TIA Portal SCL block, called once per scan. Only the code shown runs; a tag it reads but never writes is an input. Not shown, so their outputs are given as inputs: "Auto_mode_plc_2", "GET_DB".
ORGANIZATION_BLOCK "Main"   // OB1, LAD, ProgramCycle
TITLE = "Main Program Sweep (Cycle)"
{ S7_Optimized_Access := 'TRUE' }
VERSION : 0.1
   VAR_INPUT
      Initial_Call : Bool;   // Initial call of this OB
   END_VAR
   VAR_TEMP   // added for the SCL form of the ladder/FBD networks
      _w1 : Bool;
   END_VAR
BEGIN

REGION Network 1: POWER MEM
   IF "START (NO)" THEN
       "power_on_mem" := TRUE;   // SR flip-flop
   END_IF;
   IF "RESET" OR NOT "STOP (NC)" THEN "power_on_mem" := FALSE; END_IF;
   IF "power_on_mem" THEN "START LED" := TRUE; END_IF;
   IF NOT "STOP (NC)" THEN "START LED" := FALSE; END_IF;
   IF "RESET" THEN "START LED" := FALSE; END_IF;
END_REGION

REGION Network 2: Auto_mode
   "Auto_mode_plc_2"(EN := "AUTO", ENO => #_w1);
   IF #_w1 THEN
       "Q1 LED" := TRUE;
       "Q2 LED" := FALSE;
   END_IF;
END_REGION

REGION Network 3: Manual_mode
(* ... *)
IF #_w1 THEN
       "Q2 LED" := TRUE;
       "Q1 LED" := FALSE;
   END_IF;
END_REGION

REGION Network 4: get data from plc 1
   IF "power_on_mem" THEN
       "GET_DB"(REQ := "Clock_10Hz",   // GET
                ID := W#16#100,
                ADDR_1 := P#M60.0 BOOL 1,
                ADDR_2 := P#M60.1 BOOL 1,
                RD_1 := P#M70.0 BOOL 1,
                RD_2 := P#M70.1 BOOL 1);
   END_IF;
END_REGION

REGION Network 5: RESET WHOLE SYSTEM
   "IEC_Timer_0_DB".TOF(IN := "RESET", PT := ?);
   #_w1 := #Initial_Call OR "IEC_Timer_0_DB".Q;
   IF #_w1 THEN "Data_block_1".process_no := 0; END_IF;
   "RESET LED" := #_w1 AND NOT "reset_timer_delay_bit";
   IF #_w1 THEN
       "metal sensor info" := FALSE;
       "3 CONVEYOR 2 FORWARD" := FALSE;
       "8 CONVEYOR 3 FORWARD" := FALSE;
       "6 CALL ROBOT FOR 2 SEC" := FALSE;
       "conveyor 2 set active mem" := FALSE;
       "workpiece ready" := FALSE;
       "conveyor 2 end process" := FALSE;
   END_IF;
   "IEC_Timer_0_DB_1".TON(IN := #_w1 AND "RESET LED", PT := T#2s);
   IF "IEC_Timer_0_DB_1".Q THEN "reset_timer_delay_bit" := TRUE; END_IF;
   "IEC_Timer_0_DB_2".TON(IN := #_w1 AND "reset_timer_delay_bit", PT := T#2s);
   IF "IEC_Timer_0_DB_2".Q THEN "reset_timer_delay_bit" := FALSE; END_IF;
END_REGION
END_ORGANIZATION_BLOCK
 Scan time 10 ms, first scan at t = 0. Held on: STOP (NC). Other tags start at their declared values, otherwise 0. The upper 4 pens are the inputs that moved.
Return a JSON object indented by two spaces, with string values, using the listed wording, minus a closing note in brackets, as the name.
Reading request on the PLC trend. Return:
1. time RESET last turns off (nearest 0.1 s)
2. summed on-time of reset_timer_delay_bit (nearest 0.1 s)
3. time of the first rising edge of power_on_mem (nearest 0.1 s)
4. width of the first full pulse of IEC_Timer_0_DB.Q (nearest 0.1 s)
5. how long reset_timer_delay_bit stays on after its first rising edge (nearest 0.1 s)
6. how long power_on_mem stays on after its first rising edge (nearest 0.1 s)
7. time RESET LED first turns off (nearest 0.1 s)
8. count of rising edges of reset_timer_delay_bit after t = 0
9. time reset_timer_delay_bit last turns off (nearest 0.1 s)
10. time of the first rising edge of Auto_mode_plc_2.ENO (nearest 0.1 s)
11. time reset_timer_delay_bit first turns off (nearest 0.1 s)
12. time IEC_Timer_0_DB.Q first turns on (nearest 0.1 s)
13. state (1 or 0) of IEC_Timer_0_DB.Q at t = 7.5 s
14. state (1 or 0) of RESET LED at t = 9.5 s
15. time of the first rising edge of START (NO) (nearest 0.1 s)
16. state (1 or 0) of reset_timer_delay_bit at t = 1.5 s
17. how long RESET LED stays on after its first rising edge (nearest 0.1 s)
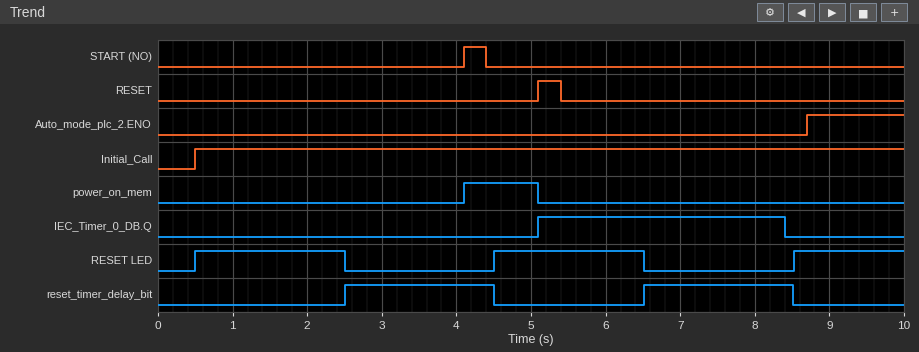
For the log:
{
  "time RESET last turns off": "5.4 s",
  "summed on-time of reset_timer_delay_bit": "4.0 s",
  "time of the first rising edge of power_on_mem": "4.1 s",
  "width of the first full pulse of IEC_Timer_0_DB.Q": "3.3 s",
  "how long reset_timer_delay_bit stays on after its first rising edge": "2.0 s",
  "how long power_on_mem stays on after its first rising edge": "1.0 s",
  "time RESET LED first turns off": "2.5 s",
  "count of rising edges of reset_timer_delay_bit after t = 0": "2",
  "time reset_timer_delay_bit last turns off": "8.5 s",
  "time of the first rising edge of Auto_mode_plc_2.ENO": "8.7 s",
  "time reset_timer_delay_bit first turns off": "4.5 s",
  "time IEC_Timer_0_DB.Q first turns on": "5.1 s",
  "state (1 or 0) of IEC_Timer_0_DB.Q at t = 7.5 s": "1",
  "state (1 or 0) of RESET LED at t = 9.5 s": "1",
  "time of the first rising edge of START (NO)": "4.1 s",
  "state (1 or 0) of reset_timer_delay_bit at t = 1.5 s": "0",
  "how long RESET LED stays on after its first rising edge": "2.0 s"
}
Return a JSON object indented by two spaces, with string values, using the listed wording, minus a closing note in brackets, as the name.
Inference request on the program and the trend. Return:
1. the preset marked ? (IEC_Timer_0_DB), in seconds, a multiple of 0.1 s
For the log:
{
  "the preset marked ? (IEC_Timer_0_DB), in seconds, a multiple of 0.1 s": "3.0 s"
}
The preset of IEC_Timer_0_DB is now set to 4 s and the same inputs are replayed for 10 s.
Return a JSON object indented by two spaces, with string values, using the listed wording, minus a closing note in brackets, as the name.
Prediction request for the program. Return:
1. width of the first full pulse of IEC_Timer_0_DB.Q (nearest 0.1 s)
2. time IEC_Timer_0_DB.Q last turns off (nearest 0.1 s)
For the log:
{
  "width of the first full pulse of IEC_Timer_0_DB.Q": "4.3 s",
  "time IEC_Timer_0_DB.Q last turns off": "9.4 s"
}
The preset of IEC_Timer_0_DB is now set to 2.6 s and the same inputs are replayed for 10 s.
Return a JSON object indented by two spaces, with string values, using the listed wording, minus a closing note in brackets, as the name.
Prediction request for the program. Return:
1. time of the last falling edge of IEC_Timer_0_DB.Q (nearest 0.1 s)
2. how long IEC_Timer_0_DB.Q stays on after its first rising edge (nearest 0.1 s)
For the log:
{
  "time of the last falling edge of IEC_Timer_0_DB.Q": "8.0 s",
  "how long IEC_Timer_0_DB.Q stays on after its first rising edge": "2.9 s"
}
